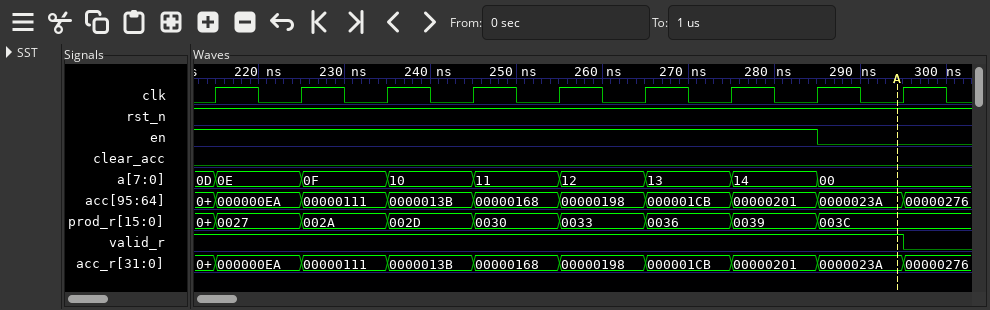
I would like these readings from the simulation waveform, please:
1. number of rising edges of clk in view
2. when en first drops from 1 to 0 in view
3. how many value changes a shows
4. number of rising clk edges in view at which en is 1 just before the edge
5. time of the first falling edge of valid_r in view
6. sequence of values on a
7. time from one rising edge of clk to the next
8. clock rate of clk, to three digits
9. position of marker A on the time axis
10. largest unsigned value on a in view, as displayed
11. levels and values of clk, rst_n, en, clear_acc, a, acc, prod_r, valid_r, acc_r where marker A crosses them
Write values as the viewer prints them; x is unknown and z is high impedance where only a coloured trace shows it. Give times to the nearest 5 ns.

9
285 ns
8
8
295 ns
0D, 0E, 0F, 10, 11, 12, 13, 14, 00
10 ns
100 MHz
295 ns
14
clk=0, rst_n=1, en=0, clear_acc=0, a=00, acc=0000023A, prod_r=003C, valid_r=1, acc_r=0000023A
